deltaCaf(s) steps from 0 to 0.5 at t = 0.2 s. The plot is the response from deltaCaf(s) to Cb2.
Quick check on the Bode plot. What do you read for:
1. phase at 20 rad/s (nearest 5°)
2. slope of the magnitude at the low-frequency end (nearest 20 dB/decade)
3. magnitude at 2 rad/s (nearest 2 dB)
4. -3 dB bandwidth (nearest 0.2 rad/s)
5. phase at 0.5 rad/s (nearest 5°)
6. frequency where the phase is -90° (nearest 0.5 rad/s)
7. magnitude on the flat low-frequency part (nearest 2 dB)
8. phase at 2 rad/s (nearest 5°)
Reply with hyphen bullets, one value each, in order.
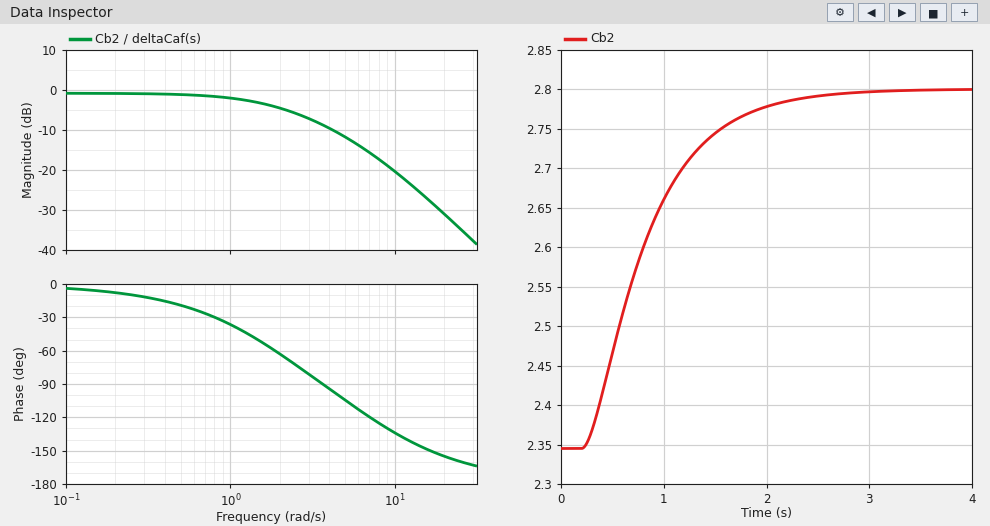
- -155°
- 0 dB/decade
- -4 dB
- 1.8 rad/s
- -20°
- 3.5 rad/s
- 0 dB
- -65°
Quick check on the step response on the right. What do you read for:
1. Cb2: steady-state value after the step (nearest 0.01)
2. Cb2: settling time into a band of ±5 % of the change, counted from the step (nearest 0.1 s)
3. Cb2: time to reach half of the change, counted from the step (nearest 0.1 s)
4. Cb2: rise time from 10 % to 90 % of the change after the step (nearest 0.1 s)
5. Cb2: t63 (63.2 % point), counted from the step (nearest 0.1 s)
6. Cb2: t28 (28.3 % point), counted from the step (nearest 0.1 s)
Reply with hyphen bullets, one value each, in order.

- 2.80
- 1.8 s
- 0.5 s
- 1.3 s
- 0.7 s
- 0.3 s
